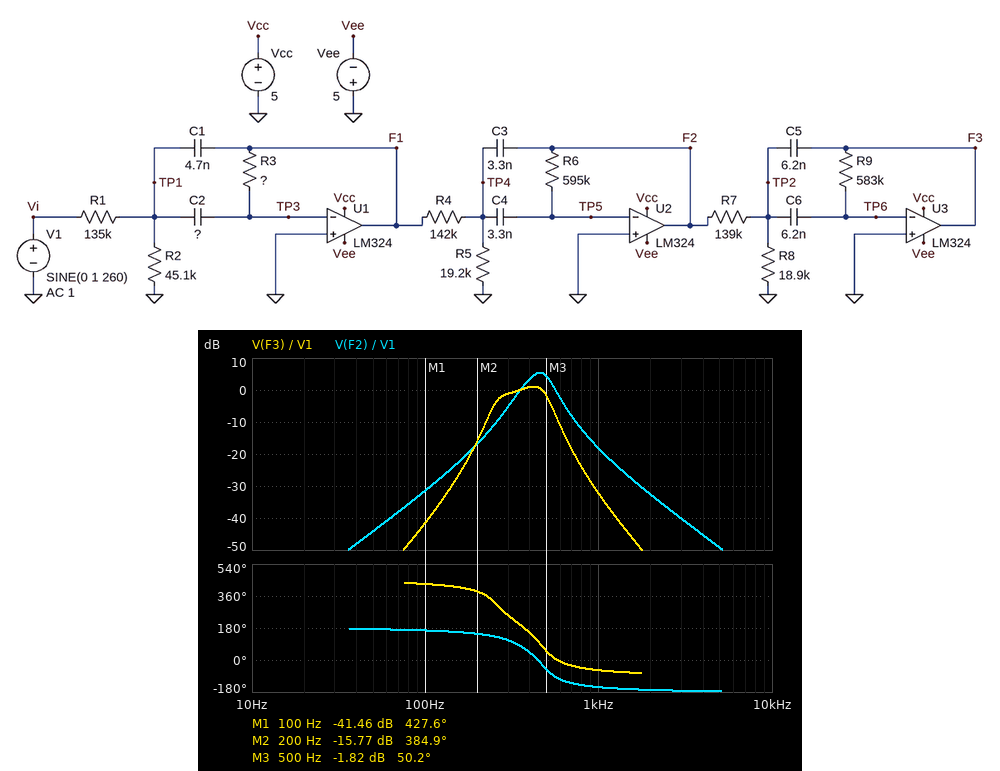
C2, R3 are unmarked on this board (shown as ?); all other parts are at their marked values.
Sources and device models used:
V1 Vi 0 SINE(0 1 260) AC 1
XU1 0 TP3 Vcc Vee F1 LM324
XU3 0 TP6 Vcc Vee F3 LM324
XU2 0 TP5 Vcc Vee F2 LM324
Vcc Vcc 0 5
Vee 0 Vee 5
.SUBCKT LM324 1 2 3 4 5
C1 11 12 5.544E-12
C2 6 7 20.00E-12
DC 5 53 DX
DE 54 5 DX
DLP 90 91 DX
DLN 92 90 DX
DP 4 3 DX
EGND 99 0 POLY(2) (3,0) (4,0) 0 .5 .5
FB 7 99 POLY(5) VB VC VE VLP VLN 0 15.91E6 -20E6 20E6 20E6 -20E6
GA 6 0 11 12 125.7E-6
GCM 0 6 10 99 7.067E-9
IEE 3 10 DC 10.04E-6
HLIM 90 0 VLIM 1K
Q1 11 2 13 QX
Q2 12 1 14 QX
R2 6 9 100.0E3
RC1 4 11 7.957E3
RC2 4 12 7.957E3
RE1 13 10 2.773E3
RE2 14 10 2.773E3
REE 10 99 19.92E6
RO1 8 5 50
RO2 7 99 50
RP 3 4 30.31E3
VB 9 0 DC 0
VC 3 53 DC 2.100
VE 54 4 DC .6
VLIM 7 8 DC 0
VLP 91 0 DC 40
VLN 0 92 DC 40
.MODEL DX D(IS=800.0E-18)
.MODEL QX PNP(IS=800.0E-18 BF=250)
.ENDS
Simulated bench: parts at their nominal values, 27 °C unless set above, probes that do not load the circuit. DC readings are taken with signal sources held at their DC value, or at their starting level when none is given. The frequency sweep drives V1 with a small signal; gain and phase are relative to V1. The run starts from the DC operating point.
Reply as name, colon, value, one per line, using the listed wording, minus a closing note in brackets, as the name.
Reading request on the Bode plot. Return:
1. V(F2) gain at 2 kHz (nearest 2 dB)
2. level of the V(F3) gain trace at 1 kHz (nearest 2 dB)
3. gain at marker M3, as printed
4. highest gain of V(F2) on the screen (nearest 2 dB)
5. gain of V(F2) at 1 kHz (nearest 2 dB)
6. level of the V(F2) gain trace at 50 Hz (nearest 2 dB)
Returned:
V(F2) gain at 2 kHz: -32 dB
level of the V(F3) gain trace at 1 kHz: -32 dB
gain at marker M3, as printed: -1.82 dB
highest gain of V(F2) on the screen: 6 dB
gain of V(F2) at 1 kHz: -18 dB
level of the V(F2) gain trace at 50 Hz: -44 dB
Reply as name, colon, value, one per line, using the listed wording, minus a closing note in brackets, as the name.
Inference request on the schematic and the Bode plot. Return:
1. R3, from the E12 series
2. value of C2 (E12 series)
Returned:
R3, from the E12 series: 390 kΩ
value of C2: 2.7 nF
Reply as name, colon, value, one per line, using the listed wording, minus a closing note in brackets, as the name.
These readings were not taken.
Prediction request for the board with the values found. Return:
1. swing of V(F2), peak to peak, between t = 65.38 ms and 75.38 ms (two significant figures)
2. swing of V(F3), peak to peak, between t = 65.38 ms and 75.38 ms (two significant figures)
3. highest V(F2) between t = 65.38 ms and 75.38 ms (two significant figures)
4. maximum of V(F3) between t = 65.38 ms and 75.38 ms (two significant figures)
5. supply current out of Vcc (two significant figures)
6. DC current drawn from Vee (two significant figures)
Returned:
swing of V(F2), peak to peak, between t = 65.38 ms and 75.38 ms: 660 mV
swing of V(F3), peak to peak, between t = 65.38 ms and 75.38 ms: 1.4 V
highest V(F2) between t = 65.38 ms and 75.38 ms: 320 mV
maximum of V(F3) between t = 65.38 ms and 75.38 ms: 680 mV
supply current out of Vcc: 1.0 mA
DC current drawn from Vee: 1.0 mA
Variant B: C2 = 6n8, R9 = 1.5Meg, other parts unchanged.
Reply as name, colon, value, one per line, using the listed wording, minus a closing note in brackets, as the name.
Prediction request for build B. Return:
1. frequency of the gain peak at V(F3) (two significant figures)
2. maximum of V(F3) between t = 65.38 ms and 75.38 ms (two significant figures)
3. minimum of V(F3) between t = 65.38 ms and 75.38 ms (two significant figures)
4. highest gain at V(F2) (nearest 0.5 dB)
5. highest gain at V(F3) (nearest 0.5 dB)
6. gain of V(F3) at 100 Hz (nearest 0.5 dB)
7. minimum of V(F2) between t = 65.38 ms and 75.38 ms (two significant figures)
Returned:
frequency of the gain peak at V(F3): 170 Hz
maximum of V(F3) between t = 65.38 ms and 75.38 ms: 970 mV
minimum of V(F3) between t = 65.38 ms and 75.38 ms: -1.0 V
highest gain at V(F2): 3.0 dB
highest gain at V(F3): 3.5 dB
gain of V(F3) at 100 Hz: -22.0 dB
minimum of V(F2) between t = 65.38 ms and 75.38 ms: -890 mV
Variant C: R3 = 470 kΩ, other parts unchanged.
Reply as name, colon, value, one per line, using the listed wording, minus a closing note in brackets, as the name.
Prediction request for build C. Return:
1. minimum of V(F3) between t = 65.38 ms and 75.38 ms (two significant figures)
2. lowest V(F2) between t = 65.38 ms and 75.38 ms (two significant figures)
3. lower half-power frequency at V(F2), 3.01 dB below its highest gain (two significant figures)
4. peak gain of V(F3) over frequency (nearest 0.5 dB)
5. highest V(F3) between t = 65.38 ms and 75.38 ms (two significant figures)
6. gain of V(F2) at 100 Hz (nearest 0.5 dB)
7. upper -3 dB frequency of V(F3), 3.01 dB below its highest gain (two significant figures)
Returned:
minimum of V(F3) between t = 65.38 ms and 75.38 ms: -940 mV
lowest V(F2) between t = 65.38 ms and 75.38 ms: -450 mV
lower half-power frequency at V(F2), 3.01 dB below its highest gain: 360 Hz
peak gain of V(F3) over frequency: 2.0 dB
highest V(F3) between t = 65.38 ms and 75.38 ms: 910 mV
gain of V(F2) at 100 Hz: -29.5 dB
upper -3 dB frequency of V(F3), 3.01 dB below its highest gain: 490 Hz
